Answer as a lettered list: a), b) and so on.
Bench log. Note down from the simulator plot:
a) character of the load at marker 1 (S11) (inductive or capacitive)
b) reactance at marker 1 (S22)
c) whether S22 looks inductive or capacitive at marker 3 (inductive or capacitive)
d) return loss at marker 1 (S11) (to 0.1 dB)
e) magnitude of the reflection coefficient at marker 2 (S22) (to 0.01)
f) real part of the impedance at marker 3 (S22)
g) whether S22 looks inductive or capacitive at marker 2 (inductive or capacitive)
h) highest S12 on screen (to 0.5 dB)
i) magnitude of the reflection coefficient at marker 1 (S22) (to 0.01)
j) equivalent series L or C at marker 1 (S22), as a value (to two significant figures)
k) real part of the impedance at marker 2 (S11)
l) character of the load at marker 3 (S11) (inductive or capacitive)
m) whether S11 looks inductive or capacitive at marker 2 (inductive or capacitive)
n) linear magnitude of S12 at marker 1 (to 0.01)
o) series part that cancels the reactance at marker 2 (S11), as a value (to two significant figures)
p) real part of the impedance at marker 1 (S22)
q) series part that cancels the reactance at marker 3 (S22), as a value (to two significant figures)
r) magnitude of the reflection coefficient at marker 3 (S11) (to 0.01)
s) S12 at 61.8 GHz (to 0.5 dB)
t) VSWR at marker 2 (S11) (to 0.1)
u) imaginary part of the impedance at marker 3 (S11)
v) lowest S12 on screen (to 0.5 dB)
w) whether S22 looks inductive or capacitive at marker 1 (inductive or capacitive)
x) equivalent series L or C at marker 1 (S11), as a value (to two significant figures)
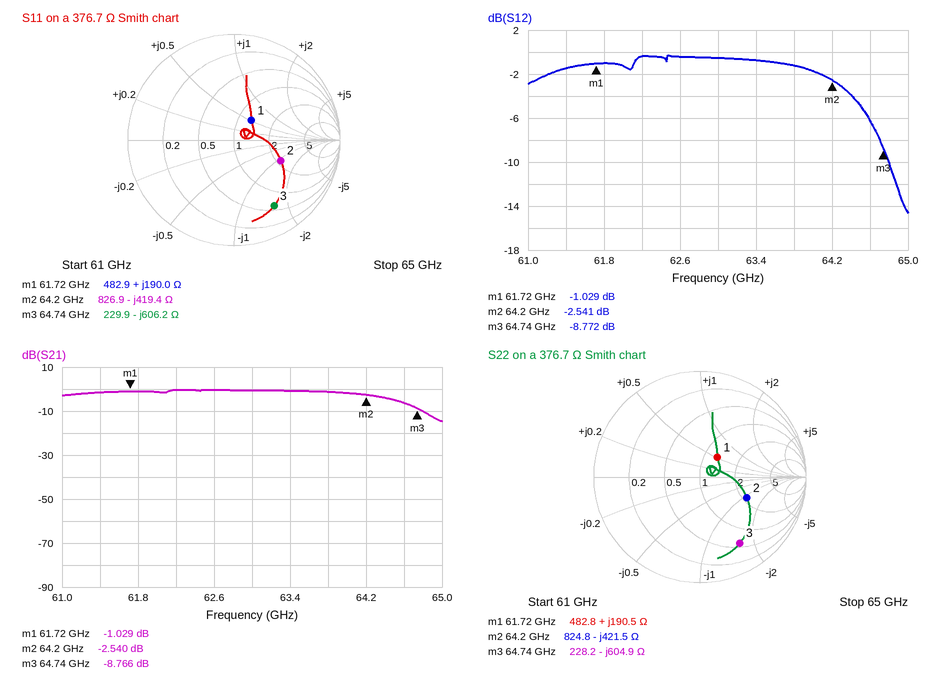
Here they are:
a) inductive
b) +190.5 Ω
c) capacitive
d) 12.1 dB
e) 0.48
f) 228.2 Ω
g) capacitive
h) -0.5 dB
i) 0.25
j) 490 pH
k) 826.9 Ω
l) capacitive
m) capacitive
n) 0.89
o) 1.0 nH
p) 482.8 Ω
q) 1.5 nH
r) 0.73
s) -1.0 dB
t) 2.9
u) -606.2 Ω
v) -14.5 dB
w) inductive
x) 490 pH
